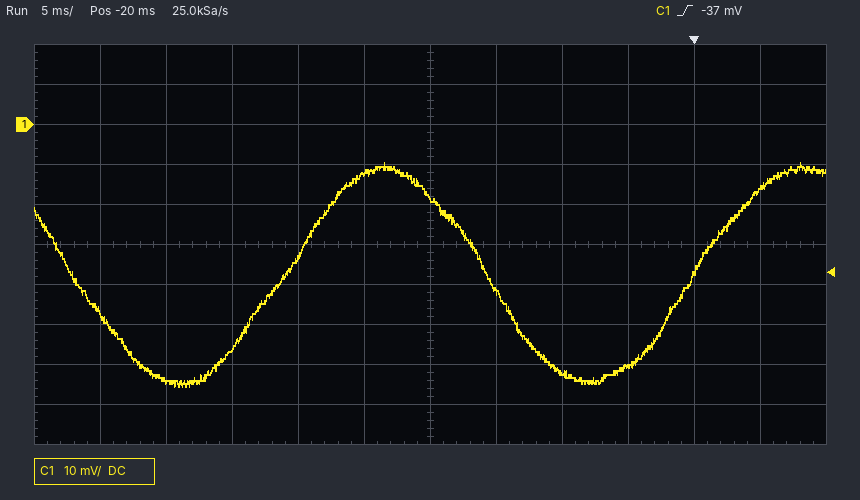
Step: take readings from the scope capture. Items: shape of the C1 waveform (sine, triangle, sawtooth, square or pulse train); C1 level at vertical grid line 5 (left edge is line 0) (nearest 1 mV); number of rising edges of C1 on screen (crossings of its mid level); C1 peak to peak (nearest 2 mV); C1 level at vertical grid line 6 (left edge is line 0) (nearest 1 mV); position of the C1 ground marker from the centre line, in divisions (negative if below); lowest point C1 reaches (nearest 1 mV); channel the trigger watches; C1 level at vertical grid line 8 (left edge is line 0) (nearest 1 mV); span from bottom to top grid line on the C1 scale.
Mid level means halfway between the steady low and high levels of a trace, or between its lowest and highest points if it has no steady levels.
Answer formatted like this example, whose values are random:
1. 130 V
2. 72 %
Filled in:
1. sine
2. -12 mV
3. 2
4. 56 mV
5. -18 mV
6. +3.0 div
7. -66 mV
8. C1
9. -62 mV
10. 100 mV
